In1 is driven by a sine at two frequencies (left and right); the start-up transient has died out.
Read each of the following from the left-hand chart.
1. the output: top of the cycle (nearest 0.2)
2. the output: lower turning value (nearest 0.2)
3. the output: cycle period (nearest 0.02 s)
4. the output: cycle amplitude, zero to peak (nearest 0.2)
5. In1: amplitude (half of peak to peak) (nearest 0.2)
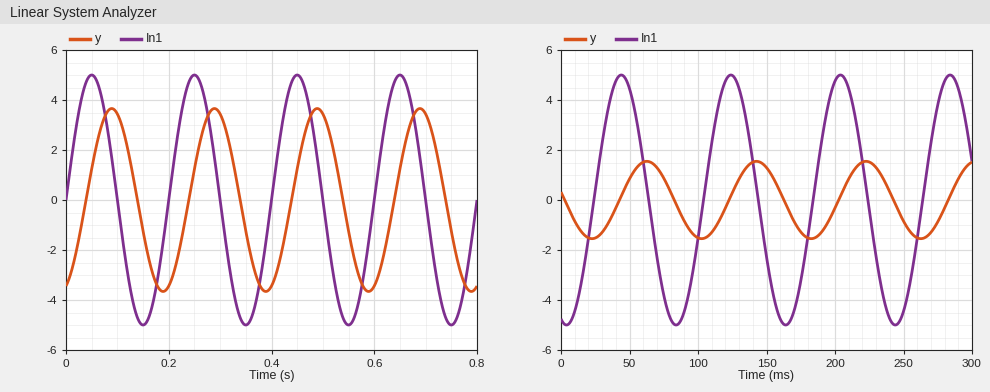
3.6
-3.6
0.20 s
3.6
5.0
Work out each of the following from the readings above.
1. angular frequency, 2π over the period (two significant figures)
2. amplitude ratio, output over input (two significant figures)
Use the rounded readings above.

31 rad/s
0.72
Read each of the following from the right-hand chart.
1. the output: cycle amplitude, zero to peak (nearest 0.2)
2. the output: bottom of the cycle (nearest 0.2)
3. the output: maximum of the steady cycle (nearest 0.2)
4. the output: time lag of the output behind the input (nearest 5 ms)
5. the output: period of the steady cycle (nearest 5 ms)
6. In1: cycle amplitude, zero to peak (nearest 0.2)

1.6
-1.6
1.6
20 ms
80 ms
5.0
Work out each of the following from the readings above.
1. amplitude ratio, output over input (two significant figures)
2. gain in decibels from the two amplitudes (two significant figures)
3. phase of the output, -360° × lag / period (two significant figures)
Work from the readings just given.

0.32
-9.9 dB
-90°
